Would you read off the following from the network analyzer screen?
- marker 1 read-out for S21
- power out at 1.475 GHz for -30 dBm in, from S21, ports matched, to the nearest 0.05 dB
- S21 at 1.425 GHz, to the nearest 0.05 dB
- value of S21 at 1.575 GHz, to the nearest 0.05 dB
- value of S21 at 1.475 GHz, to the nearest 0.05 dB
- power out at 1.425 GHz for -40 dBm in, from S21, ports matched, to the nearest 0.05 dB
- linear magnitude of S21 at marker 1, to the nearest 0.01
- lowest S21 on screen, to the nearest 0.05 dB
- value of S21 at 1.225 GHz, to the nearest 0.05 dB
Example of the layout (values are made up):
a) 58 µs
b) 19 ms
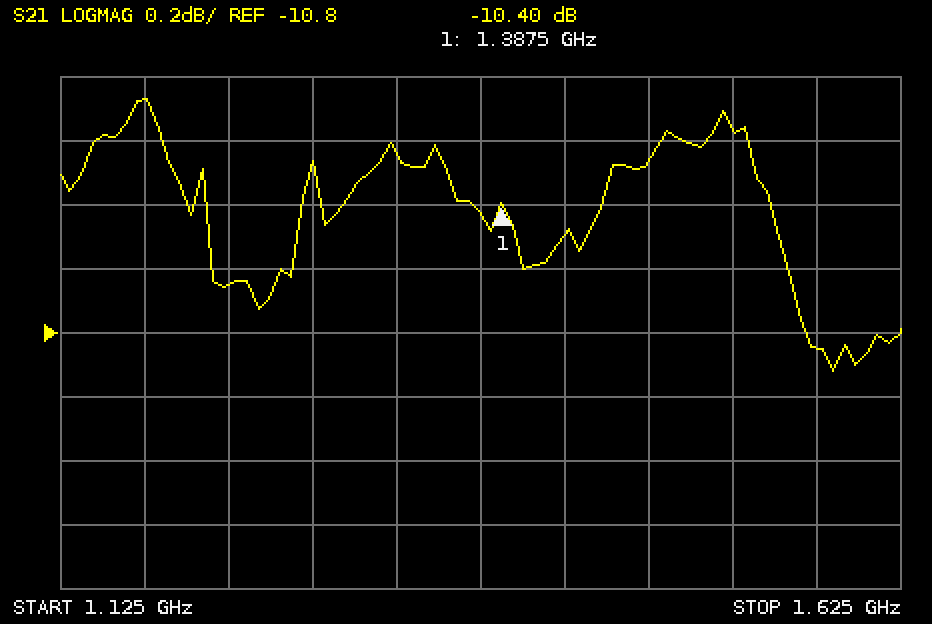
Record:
a) -10.40 dB
b) -40.25 dBm
c) -10.50 dB
d) -10.85 dB
e) -10.25 dB
f) -50.50 dBm
g) 0.30
h) -10.90 dB
i) -10.65 dB
